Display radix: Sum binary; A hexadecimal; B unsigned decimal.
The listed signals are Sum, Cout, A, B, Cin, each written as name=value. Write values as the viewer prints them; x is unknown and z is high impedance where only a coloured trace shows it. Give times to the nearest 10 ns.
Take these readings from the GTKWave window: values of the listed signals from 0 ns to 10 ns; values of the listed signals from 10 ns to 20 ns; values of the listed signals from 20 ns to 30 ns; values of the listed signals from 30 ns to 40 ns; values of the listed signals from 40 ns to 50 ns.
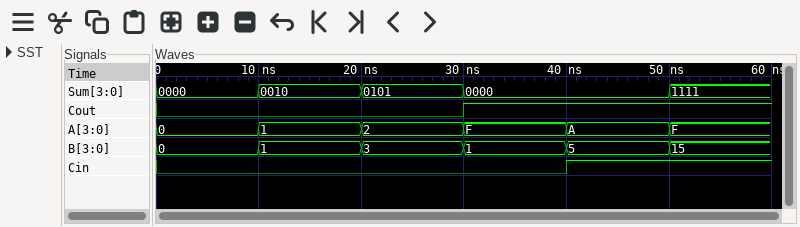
Sum=0000, Cout=0, A=0, B=0, Cin=0
Sum=0010, Cout=0, A=1, B=1, Cin=0
Sum=0101, Cout=0, A=2, B=3, Cin=0
Sum=0000, Cout=1, A=F, B=1, Cin=0
Sum=0000, Cout=1, A=A, B=5, Cin=1
